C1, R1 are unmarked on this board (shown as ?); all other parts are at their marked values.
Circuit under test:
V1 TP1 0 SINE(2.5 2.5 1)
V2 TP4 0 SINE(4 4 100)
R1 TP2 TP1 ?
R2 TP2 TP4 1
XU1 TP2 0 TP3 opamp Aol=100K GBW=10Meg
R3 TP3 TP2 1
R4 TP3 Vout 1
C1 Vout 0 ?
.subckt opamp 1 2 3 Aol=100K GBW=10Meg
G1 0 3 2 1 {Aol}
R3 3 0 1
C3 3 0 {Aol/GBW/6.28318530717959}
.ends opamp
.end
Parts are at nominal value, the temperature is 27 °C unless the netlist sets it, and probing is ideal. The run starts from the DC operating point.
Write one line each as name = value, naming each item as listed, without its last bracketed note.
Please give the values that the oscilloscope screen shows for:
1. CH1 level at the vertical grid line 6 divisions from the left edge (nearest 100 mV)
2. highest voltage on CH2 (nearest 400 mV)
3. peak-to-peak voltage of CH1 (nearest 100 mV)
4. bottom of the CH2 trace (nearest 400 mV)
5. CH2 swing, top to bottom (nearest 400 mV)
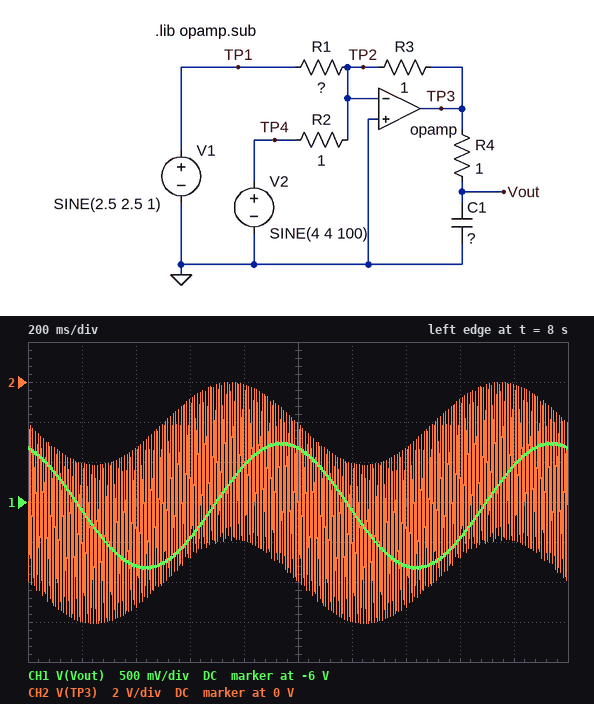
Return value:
CH1 level at the vertical grid line 6 divisions from the left edge = -6.1 V
highest voltage on CH2 = 0 V
peak-to-peak voltage of CH1 = 1.6 V
bottom of the CH2 trace = -12.0 V
CH2 swing, top to bottom = 12.0 V
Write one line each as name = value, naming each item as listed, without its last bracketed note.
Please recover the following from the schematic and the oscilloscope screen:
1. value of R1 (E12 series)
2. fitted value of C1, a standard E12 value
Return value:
value of R1 = 1.2 Ω
fitted value of C1, a standard E12 value = 390 mF
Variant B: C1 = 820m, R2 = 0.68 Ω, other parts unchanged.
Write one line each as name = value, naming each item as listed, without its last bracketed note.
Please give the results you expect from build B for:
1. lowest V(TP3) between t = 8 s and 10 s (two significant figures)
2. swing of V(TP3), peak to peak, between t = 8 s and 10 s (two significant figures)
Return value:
lowest V(TP3) between t = 8 s and 10 s = -16 V
swing of V(TP3), peak to peak, between t = 8 s and 10 s = 16 V
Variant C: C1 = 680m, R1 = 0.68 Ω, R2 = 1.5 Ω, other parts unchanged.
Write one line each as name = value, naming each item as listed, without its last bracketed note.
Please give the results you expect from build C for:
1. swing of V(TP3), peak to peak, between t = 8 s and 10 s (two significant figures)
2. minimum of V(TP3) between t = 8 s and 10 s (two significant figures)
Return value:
swing of V(TP3), peak to peak, between t = 8 s and 10 s = 13 V
minimum of V(TP3) between t = 8 s and 10 s = -13 V
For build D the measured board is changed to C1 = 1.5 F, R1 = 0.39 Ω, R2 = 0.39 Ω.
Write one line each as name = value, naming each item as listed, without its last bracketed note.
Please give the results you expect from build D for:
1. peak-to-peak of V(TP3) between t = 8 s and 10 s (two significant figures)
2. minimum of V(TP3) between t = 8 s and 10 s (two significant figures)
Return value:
peak-to-peak of V(TP3) between t = 8 s and 10 s = 33 V
minimum of V(TP3) between t = 8 s and 10 s = -33 V
